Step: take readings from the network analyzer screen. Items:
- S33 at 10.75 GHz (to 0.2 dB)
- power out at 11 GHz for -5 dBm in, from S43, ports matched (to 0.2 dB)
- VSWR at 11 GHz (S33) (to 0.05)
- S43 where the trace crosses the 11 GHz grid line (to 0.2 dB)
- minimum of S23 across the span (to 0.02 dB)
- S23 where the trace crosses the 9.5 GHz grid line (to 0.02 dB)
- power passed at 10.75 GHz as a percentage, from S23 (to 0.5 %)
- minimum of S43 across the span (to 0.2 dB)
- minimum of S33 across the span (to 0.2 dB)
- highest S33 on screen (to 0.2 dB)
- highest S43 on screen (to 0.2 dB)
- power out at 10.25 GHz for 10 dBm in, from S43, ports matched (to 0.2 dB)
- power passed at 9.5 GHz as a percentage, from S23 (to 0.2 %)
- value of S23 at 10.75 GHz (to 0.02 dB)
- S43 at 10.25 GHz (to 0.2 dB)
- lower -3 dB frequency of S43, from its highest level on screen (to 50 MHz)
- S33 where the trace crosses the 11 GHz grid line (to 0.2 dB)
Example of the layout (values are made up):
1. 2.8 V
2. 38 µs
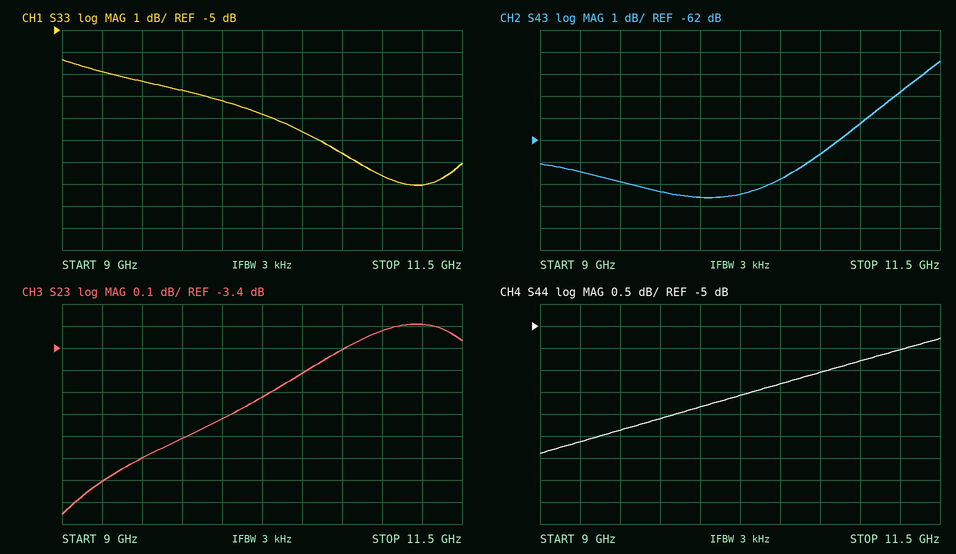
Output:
1. -10.6 dB
2. -66.2 dBm
3. 1.70
4. -61.2 dB
5. -4.16 dB
6. -3.90 dB
7. 45.5 %
8. -64.6 dB
9. -12.0 dB
10. -6.4 dB
11. -58.4 dB
12. -54.4 dBm
13. 40.8 %
14. -3.40 dB
15. -64.4 dB
16. 10.95 GHz
17. -11.6 dB
